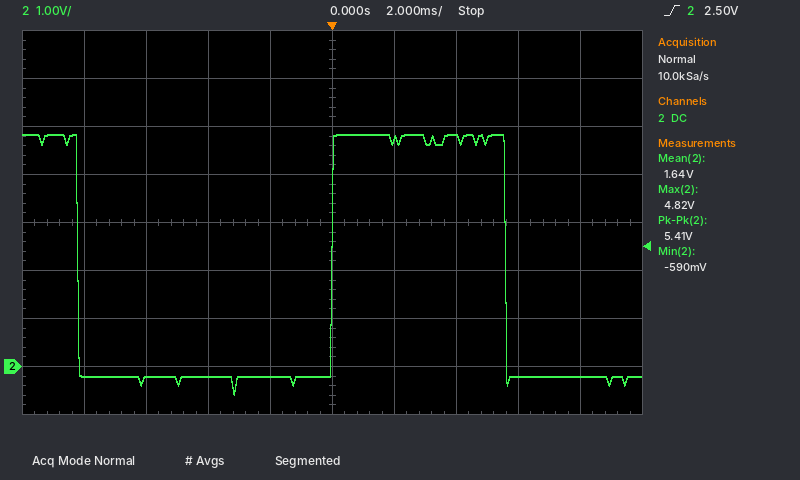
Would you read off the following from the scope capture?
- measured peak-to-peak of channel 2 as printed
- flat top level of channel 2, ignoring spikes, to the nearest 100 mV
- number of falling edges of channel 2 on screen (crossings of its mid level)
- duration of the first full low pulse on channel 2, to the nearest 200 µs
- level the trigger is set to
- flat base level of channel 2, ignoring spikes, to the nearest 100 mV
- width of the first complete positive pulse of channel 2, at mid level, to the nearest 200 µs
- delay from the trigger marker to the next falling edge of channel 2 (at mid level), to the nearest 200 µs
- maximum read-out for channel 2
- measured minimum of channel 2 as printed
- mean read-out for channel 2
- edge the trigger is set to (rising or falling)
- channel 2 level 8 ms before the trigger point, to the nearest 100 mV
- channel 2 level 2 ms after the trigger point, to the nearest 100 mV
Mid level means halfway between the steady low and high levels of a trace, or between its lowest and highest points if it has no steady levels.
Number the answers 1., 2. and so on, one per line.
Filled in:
1. 5.41 V
2. 4.8 V
3. 2
4. 8.2 ms
5. 2.50 V
6. -200 mV
7. 5.6 ms
8. 5.6 ms
9. 4.82 V
10. -590 mV
11. 1.64 V
12. rising
13. -200 mV
14. 4.7 V
